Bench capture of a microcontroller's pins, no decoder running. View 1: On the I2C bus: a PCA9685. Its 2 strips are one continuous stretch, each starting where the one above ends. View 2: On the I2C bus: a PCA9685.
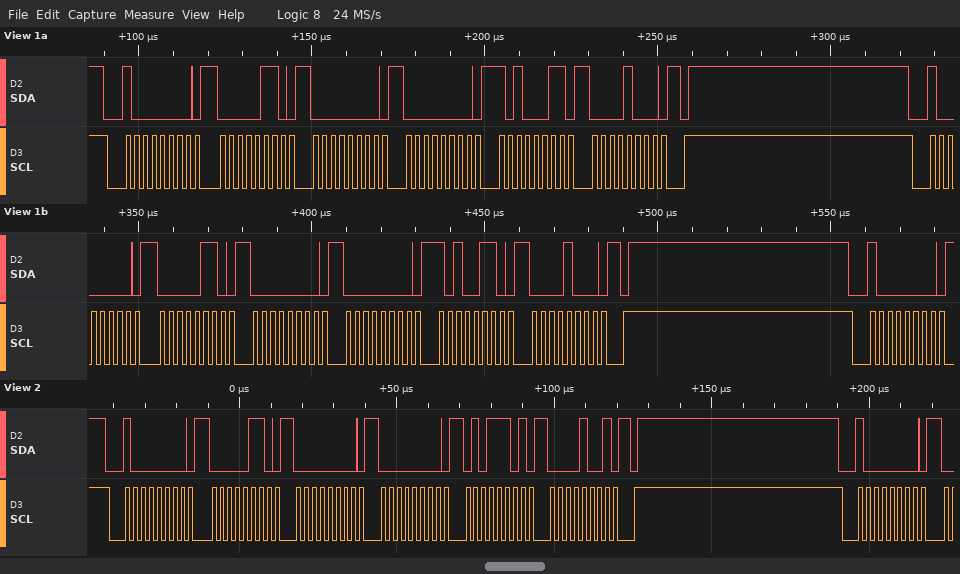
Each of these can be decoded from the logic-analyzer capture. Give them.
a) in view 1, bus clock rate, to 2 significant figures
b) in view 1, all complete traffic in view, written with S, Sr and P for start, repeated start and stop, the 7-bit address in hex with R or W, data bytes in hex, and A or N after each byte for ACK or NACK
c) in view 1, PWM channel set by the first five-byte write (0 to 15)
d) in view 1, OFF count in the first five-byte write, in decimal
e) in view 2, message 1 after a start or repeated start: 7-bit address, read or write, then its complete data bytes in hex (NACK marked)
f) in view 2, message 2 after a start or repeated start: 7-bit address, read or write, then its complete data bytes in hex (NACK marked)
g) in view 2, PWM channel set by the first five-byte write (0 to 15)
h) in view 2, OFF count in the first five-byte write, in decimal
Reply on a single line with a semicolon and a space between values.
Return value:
400 kHz; S 40W A 06 A 00 A 00 A A3 A 08 A P S 40W A 06 A 00 A 00 A A6 A 08 A P S 40W A; 0; 2211; 0x40 write: 06 00 00 5D 09; 0x40 write; 0; 2397
